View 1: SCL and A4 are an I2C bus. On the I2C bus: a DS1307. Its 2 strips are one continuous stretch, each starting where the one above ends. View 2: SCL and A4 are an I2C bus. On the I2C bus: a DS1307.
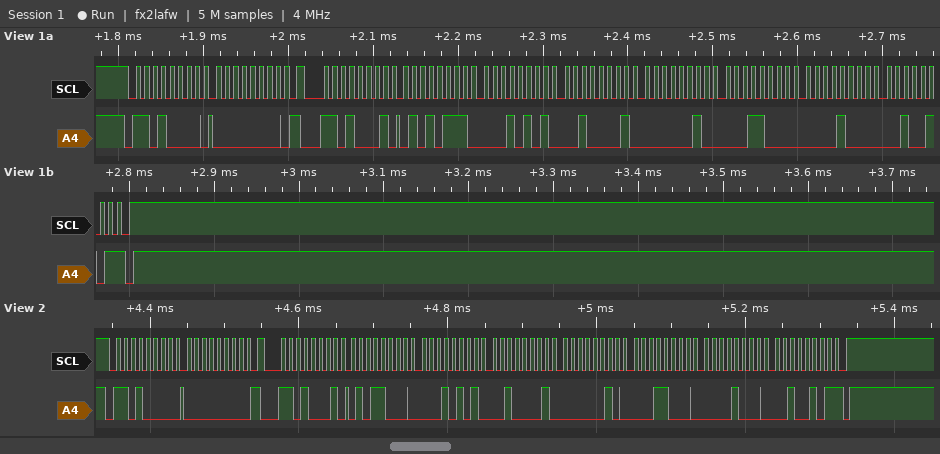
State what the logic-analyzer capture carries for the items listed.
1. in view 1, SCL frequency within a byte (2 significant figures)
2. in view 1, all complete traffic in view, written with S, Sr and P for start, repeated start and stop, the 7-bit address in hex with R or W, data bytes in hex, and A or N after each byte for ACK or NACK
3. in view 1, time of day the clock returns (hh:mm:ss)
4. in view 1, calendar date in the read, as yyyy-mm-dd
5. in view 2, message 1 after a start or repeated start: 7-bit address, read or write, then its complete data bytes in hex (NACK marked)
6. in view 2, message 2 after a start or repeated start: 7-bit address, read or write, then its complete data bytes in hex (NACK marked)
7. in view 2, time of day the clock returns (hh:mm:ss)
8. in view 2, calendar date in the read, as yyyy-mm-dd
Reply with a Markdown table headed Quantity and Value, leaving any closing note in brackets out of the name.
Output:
| Quantity | Value |
|---|---|
| in view 1, SCL frequency within a byte | 100 kHz |
| in view 1, all complete traffic in view, written with S, Sr and P for start, repeated start and stop, the 7-bit address in hex with R or W, data bytes in hex, and A or N after each byte for ACK or NACK | S 68W A 00 A Sr 68R A 57 A 15 A 21 A 02 A 18 A 08 A 25 N P |
| in view 1, time of day the clock returns | 21:15:57 |
| in view 1, calendar date in the read, as yyyy-mm-dd | 2025-08-18 |
| in view 2, message 1 after a start or repeated start: 7-bit address, read or write, then its complete data bytes in hex | 0x68 write: 00 |
| in view 2, message 2 after a start or repeated start: 7-bit address, read or write, then its complete data bytes in hex | 0x68 read: 58 15 21 02 18 08 25 NACK |
| in view 2, time of day the clock returns | 21:15:58 |
| in view 2, calendar date in the read, as yyyy-mm-dd | 2025-08-18 |
